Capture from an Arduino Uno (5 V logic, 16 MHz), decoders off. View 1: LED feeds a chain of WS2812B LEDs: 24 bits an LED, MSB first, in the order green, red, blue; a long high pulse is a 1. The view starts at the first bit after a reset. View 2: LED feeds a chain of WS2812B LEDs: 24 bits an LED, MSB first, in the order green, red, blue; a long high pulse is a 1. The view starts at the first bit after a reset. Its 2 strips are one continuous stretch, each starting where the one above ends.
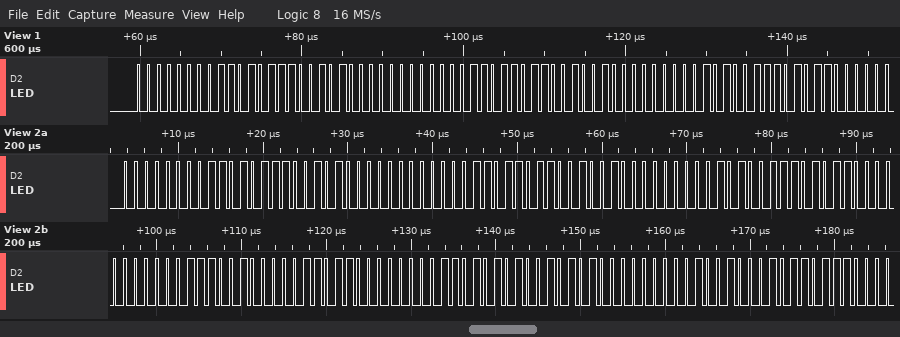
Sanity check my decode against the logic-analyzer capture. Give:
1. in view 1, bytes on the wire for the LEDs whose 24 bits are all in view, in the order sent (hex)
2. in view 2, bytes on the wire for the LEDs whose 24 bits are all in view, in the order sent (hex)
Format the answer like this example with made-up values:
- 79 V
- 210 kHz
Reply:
- 00 D7 28 00 6D 92 00 A7 58
- 00 D7 28 00 6D 92 00 A7 58 00 E4 1B 00 D5 2A 00 91 6E
